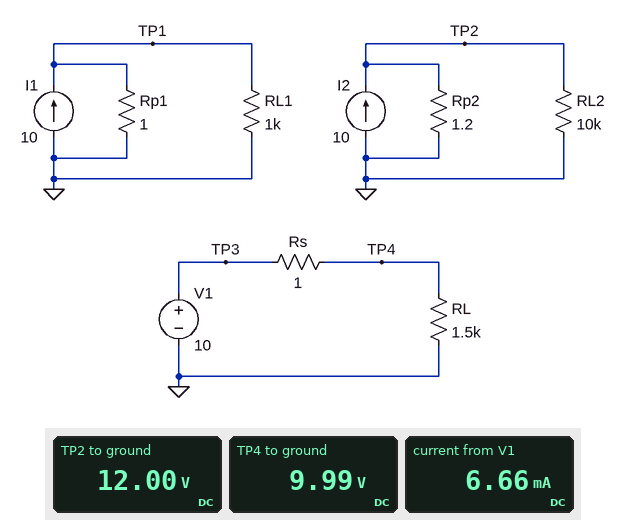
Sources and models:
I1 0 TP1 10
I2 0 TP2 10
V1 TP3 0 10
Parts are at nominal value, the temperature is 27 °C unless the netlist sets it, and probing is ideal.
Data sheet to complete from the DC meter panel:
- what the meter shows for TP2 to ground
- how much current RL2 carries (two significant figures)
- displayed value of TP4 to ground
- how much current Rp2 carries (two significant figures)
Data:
12.00 V
1.2 mA
9.99 V
10 A
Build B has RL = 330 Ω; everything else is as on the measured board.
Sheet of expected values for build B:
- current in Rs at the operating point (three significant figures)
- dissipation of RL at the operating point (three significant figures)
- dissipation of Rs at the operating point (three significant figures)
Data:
30.2 mA
301 mW
913 µW
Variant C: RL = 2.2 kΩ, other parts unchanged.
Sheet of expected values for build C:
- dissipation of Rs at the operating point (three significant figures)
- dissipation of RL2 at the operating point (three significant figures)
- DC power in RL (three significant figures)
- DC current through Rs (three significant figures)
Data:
20.6 µW
14.4 mW
45.4 mW
4.54 mA
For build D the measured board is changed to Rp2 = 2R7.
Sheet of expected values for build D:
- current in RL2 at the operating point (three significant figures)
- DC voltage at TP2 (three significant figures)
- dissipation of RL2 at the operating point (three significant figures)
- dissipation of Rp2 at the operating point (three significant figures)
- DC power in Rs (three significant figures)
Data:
2.70 mA
27.0 V
72.9 mW
270 W
44.4 µW
